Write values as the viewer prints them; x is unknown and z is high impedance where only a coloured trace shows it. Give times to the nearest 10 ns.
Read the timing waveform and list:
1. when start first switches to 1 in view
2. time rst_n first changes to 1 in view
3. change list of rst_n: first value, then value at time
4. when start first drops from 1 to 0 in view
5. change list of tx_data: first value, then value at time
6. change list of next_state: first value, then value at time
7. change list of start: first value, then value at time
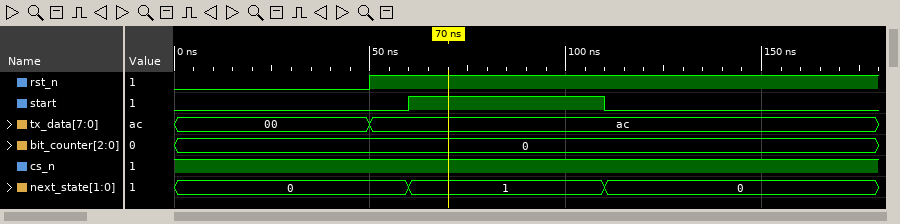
60 ns
50 ns
0, 1 at 50 ns
110 ns
00, ac at 50 ns
0, 1 at 60 ns, 0 at 110 ns
0, 1 at 60 ns, 0 at 110 ns
